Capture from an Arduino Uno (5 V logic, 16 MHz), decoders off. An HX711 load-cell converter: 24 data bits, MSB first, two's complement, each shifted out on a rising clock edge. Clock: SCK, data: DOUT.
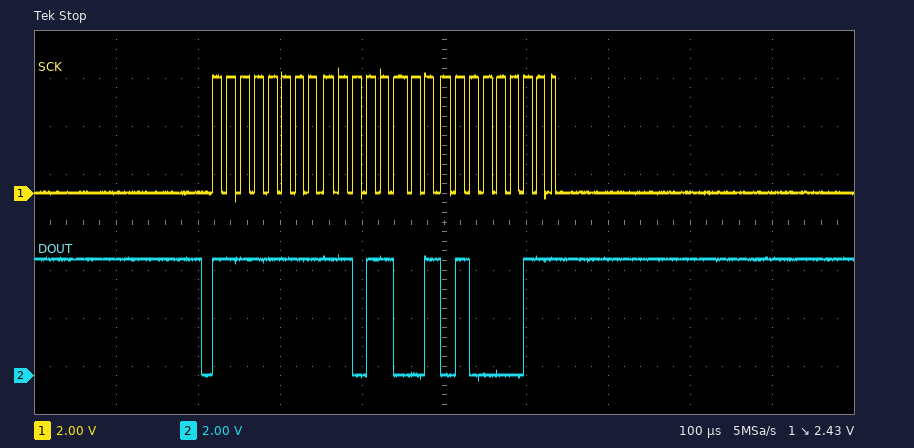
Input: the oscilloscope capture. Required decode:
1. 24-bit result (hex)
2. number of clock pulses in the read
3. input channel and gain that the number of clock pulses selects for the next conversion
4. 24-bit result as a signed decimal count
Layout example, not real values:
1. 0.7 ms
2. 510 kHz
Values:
1. 0xFFD943
2. 25
3. channel A, gain 128
4. -9917
